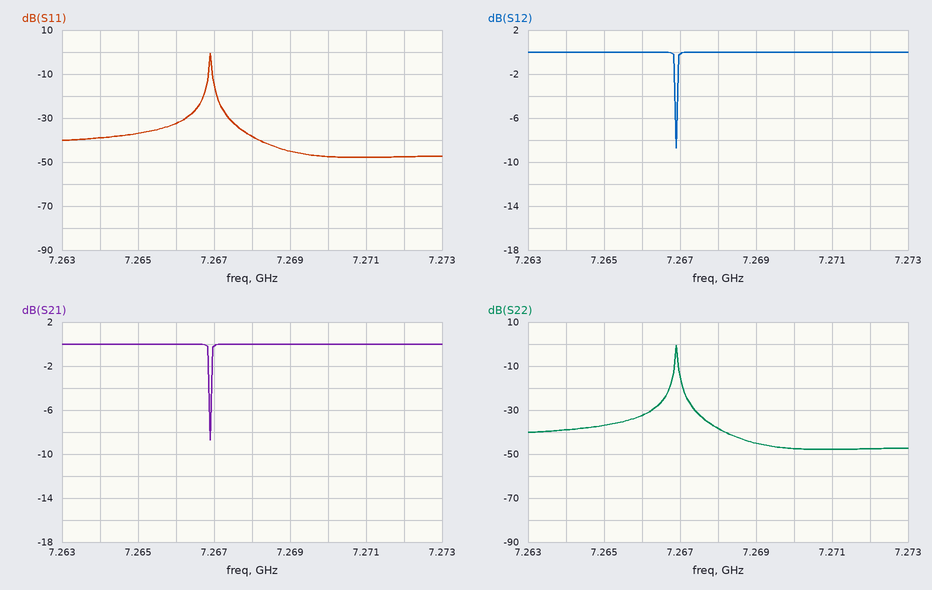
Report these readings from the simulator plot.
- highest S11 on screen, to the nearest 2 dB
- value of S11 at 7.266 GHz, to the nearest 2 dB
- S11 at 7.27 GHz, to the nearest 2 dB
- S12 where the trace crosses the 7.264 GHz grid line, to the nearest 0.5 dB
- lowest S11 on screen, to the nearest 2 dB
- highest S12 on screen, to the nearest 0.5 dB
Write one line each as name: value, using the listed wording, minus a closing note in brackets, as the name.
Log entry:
highest S11 on screen, to the nearest 2 dB: 0 dB
value of S11 at 7.266 GHz, to the nearest 2 dB: -32 dB
S11 at 7.27 GHz, to the nearest 2 dB: -48 dB
S12 where the trace crosses the 7.264 GHz grid line, to the nearest 0.5 dB: 0.0 dB
lowest S11 on screen, to the nearest 2 dB: -48 dB
highest S12 on screen, to the nearest 0.5 dB: 0.0 dB
